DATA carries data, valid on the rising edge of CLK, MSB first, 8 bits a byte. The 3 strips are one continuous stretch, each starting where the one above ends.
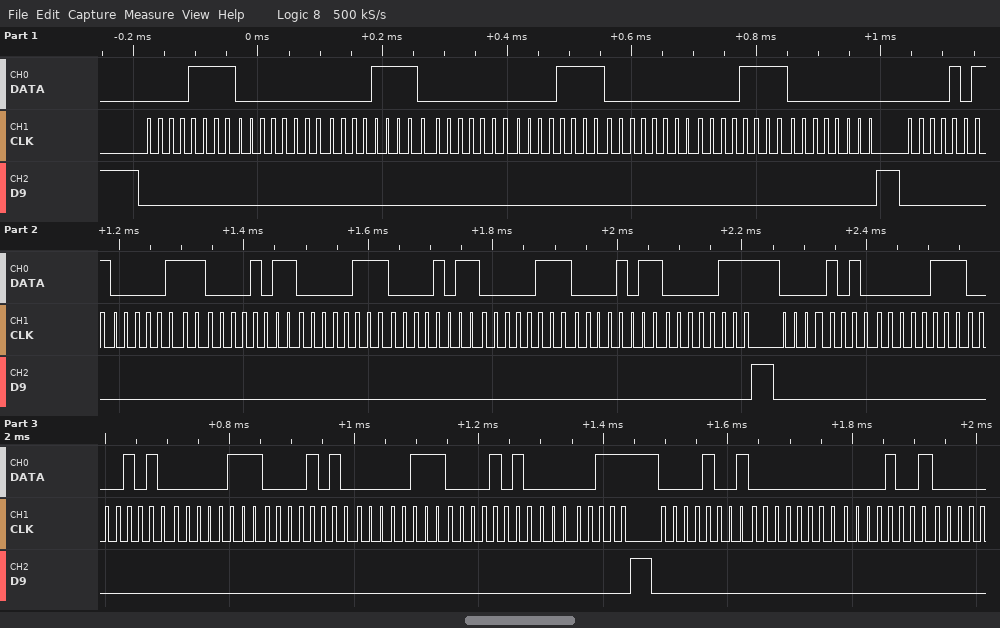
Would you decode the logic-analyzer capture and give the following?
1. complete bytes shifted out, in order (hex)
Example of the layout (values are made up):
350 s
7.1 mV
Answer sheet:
0x0F 0x00 0x0F 0x00 0x0F 0x00 0x0F 0x00 0x0B 0x07 0x0B 0x07 0x0B 0x07 0x0B 0x07 0x0A 0x07 0x0A 0x07 0x0A 0x07 0x0A 0x07 0x09 0x00 0x09
